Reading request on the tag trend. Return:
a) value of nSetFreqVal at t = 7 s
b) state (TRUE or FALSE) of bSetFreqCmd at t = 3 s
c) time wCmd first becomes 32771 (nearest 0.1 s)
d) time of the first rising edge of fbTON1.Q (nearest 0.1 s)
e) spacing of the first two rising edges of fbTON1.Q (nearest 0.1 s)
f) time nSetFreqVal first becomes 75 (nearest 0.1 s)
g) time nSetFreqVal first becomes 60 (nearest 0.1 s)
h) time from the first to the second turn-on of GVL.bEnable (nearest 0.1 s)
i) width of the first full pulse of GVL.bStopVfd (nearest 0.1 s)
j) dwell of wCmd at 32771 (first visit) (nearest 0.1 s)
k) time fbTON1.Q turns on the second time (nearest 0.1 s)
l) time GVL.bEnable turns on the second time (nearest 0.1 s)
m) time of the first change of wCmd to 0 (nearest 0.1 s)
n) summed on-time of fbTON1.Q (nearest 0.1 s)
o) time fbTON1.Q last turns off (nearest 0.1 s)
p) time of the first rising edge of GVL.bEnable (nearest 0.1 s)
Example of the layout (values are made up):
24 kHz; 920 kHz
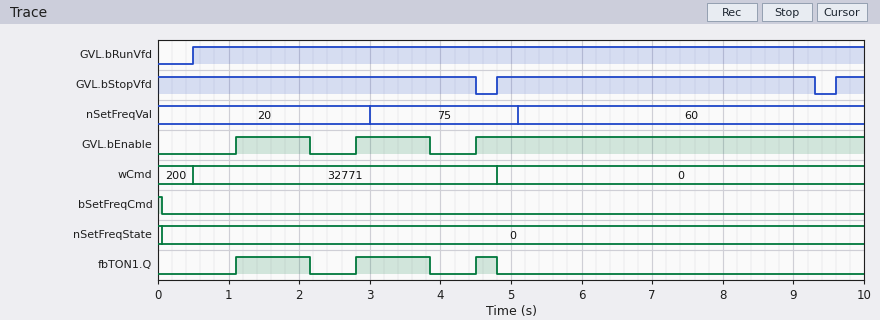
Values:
60; FALSE; 0.5 s; 1.1 s; 1.7 s; 3.0 s; 5.1 s; 1.7 s; 4.5 s; 4.3 s; 2.8 s; 2.8 s; 4.8 s; 2.4 s; 4.8 s; 1.1 s
